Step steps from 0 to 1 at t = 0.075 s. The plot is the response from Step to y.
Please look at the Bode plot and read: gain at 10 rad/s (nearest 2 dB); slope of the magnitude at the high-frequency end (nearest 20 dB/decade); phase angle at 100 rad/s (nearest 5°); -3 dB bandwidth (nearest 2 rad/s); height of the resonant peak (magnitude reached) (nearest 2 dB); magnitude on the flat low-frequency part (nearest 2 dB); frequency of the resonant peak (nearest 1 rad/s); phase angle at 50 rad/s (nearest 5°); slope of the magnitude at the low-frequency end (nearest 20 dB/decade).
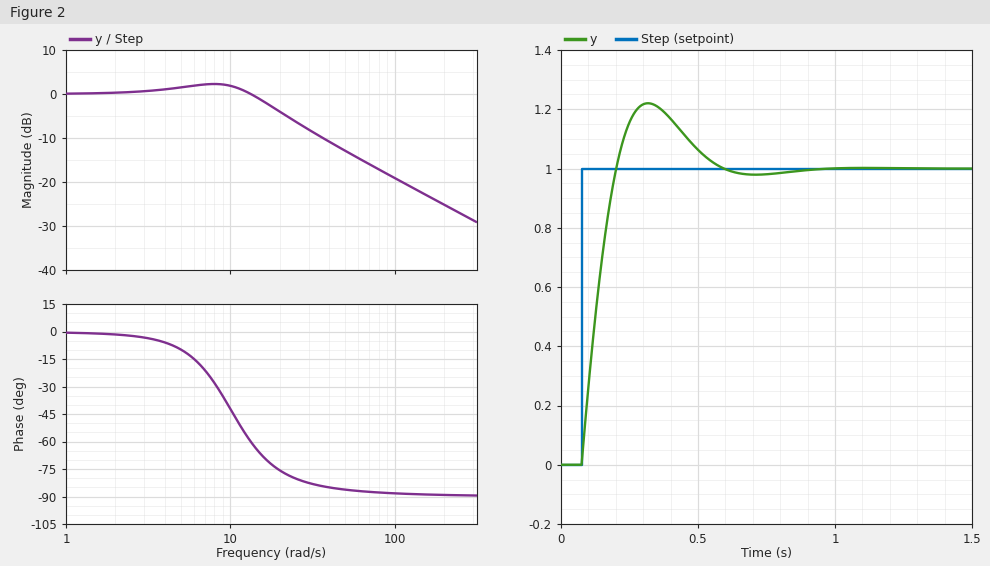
2 dB
-20 dB/decade
-90°
18 rad/s
2 dB
0 dB
8 rad/s
-85°
0 dB/decade
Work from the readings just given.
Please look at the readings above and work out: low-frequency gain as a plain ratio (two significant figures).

1.0
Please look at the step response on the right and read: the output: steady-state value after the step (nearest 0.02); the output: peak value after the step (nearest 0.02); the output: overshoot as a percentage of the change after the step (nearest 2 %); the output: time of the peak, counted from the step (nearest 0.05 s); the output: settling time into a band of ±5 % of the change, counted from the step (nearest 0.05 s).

1.00
1.22
22 %
0.25 s
0.45 s
